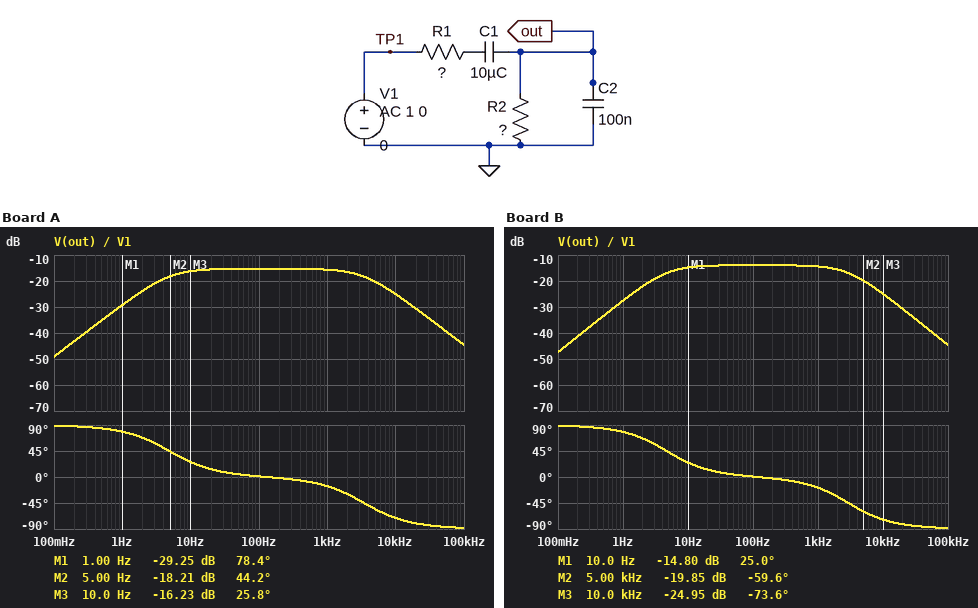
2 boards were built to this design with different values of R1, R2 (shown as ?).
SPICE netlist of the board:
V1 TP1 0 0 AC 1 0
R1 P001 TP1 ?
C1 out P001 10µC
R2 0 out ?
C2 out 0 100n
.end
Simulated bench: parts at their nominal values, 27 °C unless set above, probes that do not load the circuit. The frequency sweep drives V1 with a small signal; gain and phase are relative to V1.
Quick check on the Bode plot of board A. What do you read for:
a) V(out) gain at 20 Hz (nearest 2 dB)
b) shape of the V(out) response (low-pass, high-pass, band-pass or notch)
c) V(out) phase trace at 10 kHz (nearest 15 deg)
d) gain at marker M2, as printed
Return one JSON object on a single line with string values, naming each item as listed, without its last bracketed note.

{"V(out) gain at 20 Hz": "-16 dB", "shape of the V(out) response": "band-pass", "V(out) phase trace at 10 kHz": "-75 deg", "gain at marker M2, as printed": "-18.21 dB"}
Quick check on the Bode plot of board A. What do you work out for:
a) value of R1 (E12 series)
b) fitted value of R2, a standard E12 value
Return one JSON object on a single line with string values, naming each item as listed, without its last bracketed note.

{"value of R1": "2.7 kΩ", "fitted value of R2, a standard E12 value": "560 Ω"}
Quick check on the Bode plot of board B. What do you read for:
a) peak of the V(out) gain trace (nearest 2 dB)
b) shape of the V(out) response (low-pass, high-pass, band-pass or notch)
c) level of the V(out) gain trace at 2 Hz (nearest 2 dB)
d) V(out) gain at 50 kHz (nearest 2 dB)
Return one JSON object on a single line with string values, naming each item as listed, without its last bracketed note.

{"peak of the V(out) gain trace": "-14 dB", "shape of the V(out) response": "band-pass", "level of the V(out) gain trace at 2 Hz": "-22 dB", "V(out) gain at 50 kHz": "-38 dB"}
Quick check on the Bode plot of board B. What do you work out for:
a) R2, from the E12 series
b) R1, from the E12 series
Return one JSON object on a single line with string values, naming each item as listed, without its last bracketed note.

{"R2, from the E12 series": "680 Ω", "R1, from the E12 series": "2.7 kΩ"}
